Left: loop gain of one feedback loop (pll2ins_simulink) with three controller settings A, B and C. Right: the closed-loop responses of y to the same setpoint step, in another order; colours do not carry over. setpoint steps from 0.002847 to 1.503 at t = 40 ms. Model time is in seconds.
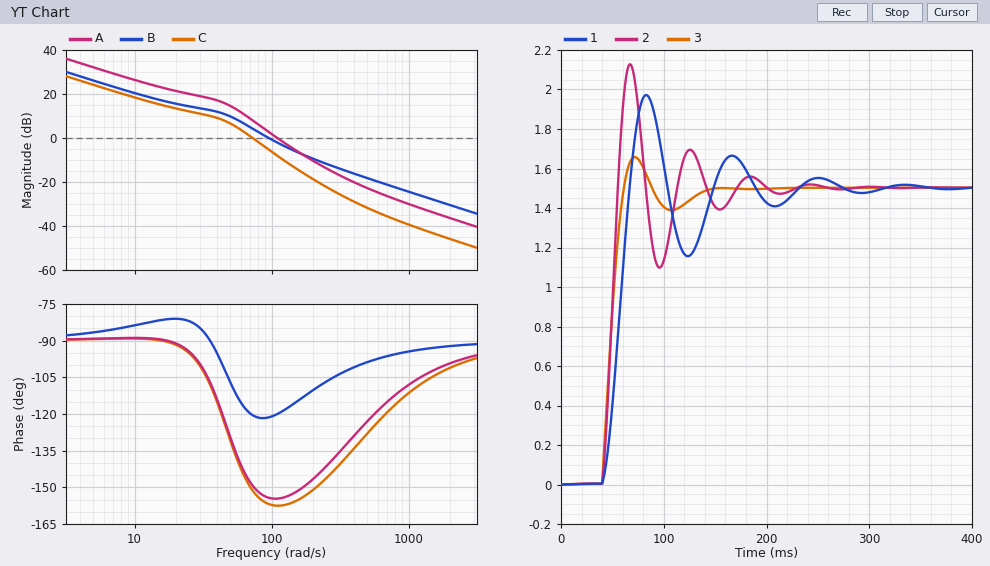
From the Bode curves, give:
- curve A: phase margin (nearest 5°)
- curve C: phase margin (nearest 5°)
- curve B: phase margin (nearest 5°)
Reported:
25°
30°
60°
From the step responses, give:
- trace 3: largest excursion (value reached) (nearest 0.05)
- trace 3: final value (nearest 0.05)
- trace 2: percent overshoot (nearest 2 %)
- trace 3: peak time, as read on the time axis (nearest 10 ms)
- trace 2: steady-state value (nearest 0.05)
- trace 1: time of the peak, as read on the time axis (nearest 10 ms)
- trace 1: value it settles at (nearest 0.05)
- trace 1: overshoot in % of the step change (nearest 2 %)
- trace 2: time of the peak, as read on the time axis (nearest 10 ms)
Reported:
1.65
1.50
42 %
70 ms
1.50
80 ms
1.50
32 %
70 ms
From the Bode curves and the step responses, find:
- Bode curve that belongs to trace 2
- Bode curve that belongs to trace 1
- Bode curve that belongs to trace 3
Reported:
A
C
B
